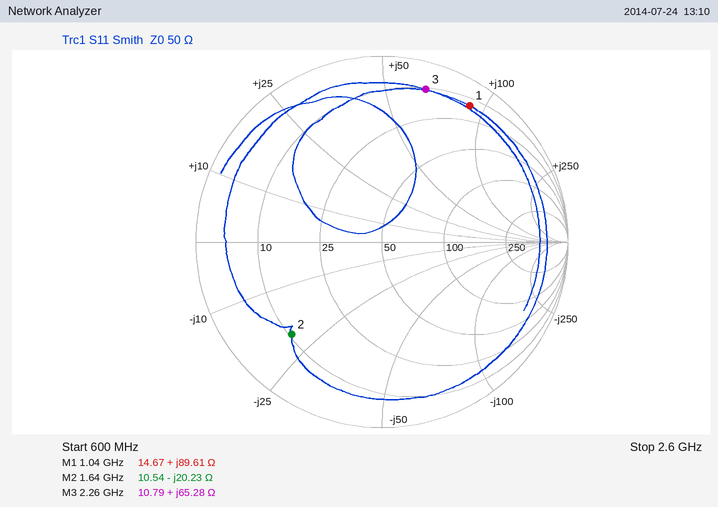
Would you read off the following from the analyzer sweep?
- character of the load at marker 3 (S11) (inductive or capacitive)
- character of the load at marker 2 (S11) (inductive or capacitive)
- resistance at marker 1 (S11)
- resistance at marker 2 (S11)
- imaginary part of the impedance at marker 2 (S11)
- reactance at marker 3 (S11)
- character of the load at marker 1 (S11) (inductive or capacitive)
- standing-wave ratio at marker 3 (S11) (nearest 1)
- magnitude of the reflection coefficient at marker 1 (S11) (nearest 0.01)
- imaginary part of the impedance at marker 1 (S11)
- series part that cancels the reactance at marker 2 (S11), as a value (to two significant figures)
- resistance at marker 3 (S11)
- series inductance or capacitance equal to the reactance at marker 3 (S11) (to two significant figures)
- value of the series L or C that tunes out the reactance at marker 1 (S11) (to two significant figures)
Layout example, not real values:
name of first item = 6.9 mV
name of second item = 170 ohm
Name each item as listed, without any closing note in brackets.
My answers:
character of the load at marker 3 (S11) = inductive
character of the load at marker 2 (S11) = capacitive
resistance at marker 1 = 14.67 Ω
resistance at marker 2 = 10.54 Ω
imaginary part of the impedance at marker 2 = -20.23 Ω
reactance at marker 3 = +65.28 Ω
character of the load at marker 1 (S11) = inductive
standing-wave ratio at marker 3 (S11) = 13
magnitude of the reflection coefficient at marker 1 (S11) = 0.87
imaginary part of the impedance at marker 1 = +89.61 Ω
series part that cancels the reactance at marker 2 (S11), as a value = 2.0 nH
resistance at marker 3 = 10.79 Ω
series inductance or capacitance equal to the reactance at marker 3 (S11) = 4.6 nH
value of the series L or C that tunes out the reactance at marker 1 (S11) = 1.7 pF
